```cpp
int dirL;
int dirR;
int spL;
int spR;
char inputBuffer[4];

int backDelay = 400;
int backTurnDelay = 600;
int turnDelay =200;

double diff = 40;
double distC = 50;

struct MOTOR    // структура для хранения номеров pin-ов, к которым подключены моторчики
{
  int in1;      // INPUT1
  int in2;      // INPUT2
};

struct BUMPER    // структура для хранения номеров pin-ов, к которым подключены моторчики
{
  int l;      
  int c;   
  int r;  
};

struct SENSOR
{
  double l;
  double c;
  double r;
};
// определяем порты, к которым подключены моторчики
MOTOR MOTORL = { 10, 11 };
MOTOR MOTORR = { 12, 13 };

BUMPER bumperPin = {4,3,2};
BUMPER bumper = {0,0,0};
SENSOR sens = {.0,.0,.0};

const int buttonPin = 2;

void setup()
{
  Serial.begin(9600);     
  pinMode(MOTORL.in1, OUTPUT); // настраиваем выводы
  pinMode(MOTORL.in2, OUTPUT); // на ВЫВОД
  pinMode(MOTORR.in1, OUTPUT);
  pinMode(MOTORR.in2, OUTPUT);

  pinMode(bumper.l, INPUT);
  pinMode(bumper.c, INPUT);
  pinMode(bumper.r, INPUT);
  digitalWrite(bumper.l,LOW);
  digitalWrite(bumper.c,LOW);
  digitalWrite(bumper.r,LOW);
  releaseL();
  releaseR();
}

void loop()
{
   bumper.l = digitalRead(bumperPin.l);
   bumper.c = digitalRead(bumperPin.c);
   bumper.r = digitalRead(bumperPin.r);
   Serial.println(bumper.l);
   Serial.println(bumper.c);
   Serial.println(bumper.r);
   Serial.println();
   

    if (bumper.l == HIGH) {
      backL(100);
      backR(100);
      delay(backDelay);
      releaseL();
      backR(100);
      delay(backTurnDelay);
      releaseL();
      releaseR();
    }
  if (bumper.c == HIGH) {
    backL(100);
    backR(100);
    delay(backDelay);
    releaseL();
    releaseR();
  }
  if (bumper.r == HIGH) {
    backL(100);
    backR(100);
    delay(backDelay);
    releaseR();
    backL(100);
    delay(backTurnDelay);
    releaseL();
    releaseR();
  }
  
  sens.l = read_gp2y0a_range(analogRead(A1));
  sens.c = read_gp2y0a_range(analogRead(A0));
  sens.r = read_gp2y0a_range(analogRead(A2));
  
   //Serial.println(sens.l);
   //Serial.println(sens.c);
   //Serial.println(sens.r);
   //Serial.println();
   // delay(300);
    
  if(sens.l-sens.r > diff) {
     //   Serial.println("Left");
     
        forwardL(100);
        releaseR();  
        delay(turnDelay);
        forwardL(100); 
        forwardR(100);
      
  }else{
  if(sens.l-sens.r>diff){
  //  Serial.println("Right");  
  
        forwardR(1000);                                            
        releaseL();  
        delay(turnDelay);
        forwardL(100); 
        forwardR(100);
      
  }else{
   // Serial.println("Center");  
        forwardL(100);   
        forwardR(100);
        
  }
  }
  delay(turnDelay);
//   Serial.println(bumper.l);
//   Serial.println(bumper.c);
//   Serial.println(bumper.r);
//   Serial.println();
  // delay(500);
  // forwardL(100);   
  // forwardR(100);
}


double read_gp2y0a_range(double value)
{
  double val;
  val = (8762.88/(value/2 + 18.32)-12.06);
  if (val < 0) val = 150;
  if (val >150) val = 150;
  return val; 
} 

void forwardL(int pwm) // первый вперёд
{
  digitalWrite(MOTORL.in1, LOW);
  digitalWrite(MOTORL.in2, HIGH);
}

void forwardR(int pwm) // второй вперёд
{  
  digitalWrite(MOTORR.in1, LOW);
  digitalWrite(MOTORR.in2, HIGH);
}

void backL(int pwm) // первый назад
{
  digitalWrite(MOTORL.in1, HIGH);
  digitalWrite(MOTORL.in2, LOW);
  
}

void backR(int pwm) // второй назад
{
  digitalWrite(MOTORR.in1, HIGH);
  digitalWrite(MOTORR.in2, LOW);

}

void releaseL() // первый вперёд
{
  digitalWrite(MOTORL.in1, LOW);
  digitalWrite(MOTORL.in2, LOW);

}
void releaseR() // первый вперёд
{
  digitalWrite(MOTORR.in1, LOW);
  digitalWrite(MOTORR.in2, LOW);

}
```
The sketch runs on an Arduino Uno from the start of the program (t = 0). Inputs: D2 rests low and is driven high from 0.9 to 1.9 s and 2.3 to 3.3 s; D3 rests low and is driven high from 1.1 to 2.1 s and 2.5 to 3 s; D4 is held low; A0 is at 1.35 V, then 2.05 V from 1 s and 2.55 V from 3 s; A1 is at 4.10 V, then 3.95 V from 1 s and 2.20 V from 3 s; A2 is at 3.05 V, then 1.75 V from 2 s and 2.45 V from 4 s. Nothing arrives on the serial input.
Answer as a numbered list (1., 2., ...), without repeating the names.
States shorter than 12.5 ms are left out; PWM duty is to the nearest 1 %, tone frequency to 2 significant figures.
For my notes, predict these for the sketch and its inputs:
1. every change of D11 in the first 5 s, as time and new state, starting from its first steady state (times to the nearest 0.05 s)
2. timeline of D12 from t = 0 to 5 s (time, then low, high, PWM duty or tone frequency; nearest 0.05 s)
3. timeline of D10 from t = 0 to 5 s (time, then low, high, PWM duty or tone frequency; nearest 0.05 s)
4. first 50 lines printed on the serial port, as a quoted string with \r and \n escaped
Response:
1. 0 s high; 1 s low; 2 s high; 2.4 s low; 3.4 s high
2. 0 s low; 1 s high; 1.4 s low; 2.4 s high; 2.8 s low
3. 0 s low; 1 s high; 2 s low; 2.4 s high; 3.4 s low
4. "0\r\n0\r\n0\r\n\r\n0\r\n0\r\n0\r\n\r\n0\r\n0\r\n0\r\n\r\n0\r\n0\r\n0\r\n\r\n0\r\n0\r\n0\r\n\r\n0\r\n0\r\n1\r\n\r\n0\r\n0\r\n0\r\n\r\n0\r\n0\r\n1\r\n\r\n0\r\n0\r\n0\r\n\r\n0\r\n0\r\n0\r\n\r\n0\r\n0\r\n0\r\n\r\n0\r\n0\r\n0\r\n\r\n0\r\n0\r\n"
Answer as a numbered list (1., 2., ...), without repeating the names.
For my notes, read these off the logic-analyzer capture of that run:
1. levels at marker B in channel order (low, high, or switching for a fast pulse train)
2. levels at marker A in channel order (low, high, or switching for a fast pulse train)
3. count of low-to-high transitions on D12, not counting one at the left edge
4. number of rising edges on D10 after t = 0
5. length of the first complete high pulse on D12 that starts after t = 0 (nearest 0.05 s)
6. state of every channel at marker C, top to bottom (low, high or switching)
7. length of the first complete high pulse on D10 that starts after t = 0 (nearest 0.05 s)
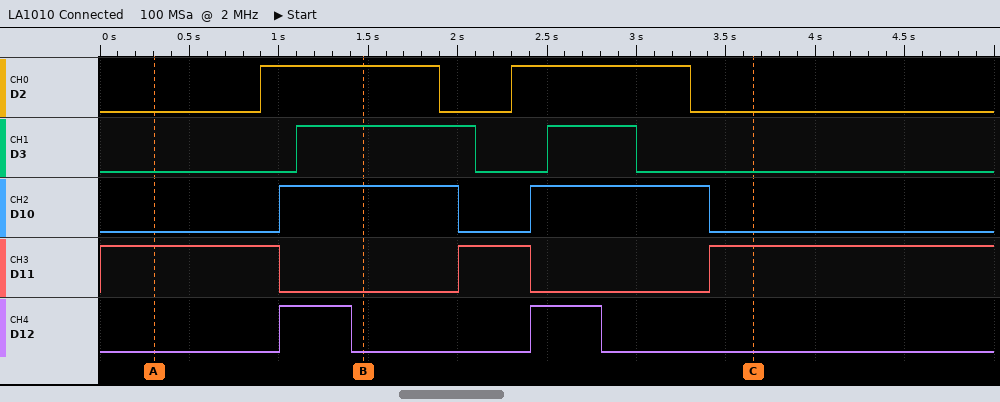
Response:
1. D2 high, D3 high, D10 high, D11 low, D12 low
2. D2 low, D3 low, D10 low, D11 high, D12 low
3. 2
4. 2
5. 0.40 s
6. D2 low, D3 low, D10 low, D11 high, D12 low
7. 1.00 s
